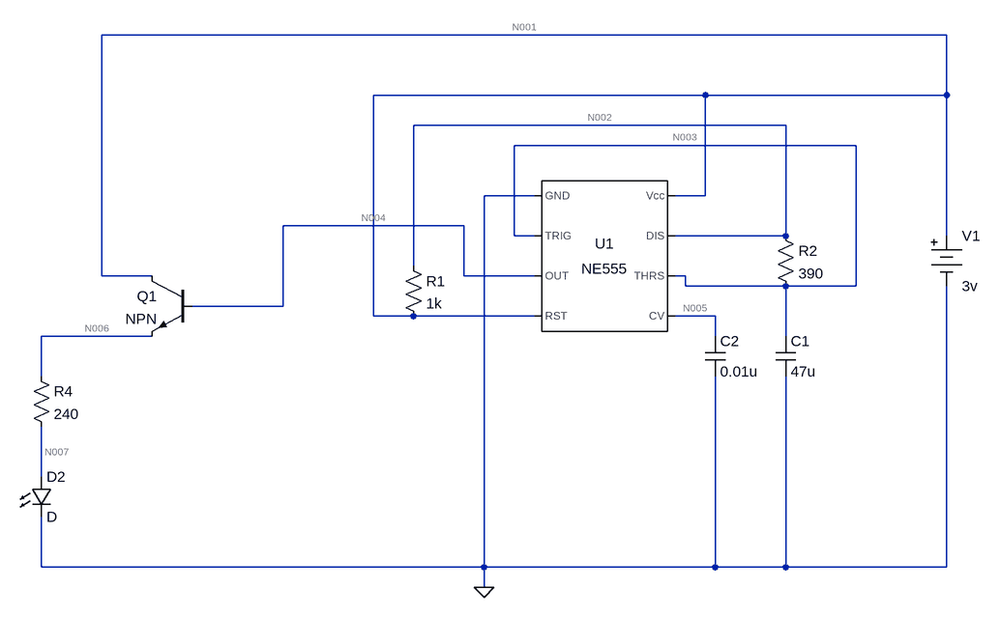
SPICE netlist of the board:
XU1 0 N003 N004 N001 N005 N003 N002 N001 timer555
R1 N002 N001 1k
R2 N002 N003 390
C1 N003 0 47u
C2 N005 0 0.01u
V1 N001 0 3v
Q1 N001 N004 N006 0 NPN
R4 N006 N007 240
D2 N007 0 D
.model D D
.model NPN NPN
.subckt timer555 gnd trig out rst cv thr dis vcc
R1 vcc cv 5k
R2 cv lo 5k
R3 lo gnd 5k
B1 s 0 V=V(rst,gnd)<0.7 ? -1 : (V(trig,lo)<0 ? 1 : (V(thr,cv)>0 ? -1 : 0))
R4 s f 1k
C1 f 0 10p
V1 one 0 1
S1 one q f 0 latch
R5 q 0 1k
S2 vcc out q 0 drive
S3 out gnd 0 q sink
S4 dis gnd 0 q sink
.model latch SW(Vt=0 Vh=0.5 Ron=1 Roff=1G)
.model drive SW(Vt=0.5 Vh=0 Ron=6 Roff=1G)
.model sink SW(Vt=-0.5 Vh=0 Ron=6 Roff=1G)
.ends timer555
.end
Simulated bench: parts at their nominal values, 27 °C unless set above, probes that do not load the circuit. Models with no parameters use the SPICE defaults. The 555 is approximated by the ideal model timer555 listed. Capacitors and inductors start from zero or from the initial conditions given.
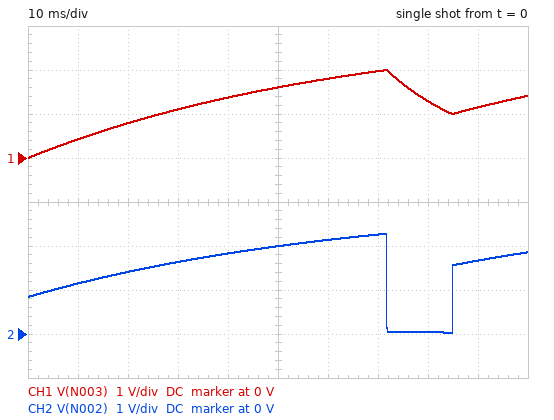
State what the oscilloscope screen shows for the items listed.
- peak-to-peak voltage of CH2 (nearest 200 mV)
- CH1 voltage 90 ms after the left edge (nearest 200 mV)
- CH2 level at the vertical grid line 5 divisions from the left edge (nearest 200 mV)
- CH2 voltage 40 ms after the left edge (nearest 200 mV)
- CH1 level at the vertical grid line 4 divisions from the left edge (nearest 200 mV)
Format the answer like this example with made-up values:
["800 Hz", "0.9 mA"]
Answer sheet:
["2.2 V", "1.2 V", "2.0 V", "1.8 V", "1.4 V"]
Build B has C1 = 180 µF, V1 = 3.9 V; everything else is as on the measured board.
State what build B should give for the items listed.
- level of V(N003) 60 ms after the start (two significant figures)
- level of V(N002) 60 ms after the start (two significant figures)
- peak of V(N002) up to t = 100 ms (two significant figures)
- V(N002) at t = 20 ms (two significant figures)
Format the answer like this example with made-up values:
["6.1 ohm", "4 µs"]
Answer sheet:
["830 mV", "1.7 V", "2.0 V", "1.3 V"]
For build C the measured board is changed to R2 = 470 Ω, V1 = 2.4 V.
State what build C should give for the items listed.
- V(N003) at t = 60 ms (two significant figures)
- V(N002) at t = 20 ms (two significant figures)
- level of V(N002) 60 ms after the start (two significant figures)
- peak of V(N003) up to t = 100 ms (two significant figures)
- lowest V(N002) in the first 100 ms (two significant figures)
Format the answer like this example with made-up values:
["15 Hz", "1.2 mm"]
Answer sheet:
["1.4 V", "1.2 V", "1.7 V", "1.6 V", "24 mV"]
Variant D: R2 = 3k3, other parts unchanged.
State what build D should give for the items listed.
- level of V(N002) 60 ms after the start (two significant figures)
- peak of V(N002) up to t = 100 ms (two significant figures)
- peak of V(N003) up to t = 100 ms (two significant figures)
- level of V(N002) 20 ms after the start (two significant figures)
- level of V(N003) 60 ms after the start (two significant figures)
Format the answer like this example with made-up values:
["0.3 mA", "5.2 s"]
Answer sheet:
["2.5 V", "2.6 V", "1.2 V", "2.4 V", "770 mV"]
